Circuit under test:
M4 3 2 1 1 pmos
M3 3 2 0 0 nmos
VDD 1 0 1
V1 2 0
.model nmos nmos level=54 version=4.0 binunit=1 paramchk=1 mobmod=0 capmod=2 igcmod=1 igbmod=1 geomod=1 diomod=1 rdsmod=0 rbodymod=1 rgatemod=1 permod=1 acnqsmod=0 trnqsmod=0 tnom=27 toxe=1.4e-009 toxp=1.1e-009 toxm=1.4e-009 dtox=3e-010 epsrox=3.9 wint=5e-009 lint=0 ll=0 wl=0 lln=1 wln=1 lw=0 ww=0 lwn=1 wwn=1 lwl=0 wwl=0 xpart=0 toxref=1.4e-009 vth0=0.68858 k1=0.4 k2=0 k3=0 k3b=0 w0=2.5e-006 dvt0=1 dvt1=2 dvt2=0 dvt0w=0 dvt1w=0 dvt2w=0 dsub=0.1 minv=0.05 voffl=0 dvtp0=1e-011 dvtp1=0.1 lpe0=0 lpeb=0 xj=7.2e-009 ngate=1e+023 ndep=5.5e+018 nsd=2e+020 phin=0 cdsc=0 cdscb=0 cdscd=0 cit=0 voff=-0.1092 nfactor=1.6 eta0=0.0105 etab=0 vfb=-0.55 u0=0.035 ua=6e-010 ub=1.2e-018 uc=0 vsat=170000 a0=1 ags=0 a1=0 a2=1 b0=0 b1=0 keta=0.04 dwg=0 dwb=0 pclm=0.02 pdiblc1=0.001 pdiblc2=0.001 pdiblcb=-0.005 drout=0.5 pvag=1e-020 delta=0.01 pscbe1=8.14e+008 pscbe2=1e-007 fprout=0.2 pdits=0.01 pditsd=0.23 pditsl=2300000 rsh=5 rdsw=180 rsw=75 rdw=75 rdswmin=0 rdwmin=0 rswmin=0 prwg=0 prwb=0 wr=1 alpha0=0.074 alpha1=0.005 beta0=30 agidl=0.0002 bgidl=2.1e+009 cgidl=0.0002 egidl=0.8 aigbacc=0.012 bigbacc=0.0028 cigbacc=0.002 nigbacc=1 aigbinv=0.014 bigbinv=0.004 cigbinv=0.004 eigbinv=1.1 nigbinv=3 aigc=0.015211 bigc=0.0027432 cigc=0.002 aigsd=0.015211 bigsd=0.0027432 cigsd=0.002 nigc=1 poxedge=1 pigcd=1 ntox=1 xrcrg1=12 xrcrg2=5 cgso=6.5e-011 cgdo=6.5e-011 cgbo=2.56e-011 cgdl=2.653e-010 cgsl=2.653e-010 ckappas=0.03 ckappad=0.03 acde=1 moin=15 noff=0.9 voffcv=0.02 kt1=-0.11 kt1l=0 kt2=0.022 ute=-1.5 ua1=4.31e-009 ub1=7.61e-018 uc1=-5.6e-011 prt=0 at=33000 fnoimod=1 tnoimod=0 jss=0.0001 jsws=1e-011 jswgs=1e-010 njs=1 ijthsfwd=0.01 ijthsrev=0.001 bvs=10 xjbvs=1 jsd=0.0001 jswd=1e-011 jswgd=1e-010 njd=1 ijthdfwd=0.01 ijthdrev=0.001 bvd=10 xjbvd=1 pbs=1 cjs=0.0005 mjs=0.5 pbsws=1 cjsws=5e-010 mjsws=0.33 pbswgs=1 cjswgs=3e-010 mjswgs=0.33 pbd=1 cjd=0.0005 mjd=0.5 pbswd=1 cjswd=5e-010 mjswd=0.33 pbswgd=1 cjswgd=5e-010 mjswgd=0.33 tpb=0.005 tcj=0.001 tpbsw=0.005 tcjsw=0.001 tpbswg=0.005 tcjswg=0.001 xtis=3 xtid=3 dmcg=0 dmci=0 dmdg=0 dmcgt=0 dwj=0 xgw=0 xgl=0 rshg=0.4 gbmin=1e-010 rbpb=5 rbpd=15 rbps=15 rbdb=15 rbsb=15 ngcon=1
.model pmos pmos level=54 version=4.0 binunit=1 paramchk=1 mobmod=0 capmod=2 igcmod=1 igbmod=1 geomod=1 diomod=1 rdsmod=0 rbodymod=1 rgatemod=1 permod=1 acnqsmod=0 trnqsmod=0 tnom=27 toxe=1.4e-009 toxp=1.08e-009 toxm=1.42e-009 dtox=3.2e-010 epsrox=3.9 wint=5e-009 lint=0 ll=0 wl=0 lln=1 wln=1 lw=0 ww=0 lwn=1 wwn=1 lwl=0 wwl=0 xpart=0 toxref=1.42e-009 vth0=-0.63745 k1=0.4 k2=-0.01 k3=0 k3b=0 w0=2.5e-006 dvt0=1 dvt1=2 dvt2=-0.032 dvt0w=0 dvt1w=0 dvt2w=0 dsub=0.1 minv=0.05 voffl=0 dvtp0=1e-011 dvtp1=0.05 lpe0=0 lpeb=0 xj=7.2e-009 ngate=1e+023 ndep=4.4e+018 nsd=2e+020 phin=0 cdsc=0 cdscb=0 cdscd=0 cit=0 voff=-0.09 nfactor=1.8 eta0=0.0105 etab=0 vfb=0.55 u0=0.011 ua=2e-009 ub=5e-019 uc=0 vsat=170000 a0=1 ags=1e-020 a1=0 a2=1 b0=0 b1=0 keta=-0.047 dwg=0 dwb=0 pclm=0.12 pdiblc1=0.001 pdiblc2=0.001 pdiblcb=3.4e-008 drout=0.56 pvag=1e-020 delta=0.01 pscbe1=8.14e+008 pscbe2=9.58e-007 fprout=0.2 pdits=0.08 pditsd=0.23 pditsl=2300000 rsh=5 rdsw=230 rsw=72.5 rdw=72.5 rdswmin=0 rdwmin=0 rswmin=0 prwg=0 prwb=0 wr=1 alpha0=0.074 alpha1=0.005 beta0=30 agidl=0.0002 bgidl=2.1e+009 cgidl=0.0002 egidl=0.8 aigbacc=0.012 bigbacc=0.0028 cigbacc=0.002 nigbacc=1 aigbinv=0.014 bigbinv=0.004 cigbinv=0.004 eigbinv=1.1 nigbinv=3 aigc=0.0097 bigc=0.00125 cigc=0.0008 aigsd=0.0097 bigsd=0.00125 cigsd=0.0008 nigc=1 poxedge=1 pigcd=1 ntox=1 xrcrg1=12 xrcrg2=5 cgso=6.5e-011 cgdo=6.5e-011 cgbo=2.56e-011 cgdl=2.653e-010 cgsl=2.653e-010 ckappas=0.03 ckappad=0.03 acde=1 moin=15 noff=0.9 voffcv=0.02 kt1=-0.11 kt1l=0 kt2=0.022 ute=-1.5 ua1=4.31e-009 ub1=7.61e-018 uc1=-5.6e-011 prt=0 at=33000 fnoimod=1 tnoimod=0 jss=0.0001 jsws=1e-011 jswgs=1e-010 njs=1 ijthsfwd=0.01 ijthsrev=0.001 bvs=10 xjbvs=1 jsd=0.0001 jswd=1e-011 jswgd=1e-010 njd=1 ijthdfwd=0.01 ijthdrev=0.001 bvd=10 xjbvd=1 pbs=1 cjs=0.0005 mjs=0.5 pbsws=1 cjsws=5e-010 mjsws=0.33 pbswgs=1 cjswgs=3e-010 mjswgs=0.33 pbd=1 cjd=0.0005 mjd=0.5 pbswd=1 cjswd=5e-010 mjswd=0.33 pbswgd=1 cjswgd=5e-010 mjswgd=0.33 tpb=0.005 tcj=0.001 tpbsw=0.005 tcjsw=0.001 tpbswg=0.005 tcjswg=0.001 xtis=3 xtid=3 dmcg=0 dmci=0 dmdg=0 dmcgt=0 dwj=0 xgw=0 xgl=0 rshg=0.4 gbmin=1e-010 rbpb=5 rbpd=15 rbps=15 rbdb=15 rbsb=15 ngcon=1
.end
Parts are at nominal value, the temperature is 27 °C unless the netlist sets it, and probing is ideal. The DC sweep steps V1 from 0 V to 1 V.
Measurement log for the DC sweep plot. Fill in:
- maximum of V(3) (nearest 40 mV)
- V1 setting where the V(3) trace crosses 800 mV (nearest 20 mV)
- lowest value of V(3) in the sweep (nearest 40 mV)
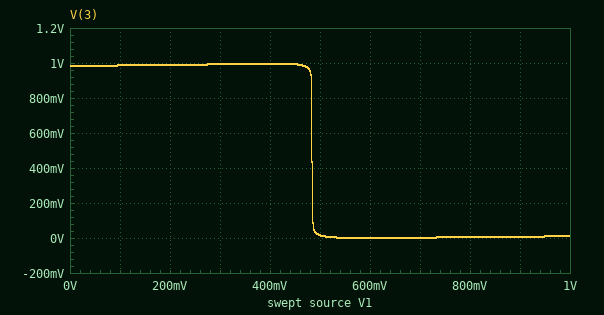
1.00 V
480 mV
0 V
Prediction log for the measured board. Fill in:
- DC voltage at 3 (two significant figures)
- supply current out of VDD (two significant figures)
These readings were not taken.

980 mV
950 nA
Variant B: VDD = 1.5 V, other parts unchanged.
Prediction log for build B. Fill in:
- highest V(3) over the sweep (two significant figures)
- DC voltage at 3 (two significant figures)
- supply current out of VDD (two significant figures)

1.5 V
1.4 V
13 µA
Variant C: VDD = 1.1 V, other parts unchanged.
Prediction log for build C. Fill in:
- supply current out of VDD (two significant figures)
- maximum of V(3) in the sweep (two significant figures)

1.6 µA
1.1 V
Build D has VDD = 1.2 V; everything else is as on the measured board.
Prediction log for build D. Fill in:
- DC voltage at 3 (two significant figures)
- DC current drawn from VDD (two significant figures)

1.2 V
2.7 µA
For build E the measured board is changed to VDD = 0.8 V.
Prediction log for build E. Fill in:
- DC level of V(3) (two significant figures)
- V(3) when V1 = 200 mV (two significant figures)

790 mV
800 mV
